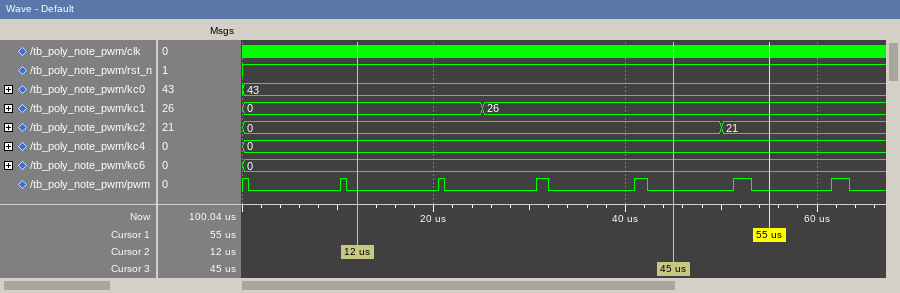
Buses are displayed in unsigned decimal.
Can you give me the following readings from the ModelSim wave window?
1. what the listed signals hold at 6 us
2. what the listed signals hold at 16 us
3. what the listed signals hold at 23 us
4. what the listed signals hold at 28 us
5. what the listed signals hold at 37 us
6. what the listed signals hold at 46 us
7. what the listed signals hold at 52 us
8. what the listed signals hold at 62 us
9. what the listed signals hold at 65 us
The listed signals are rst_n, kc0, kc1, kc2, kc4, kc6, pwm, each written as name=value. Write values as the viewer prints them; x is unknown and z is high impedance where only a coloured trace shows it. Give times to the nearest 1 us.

rst_n=1, kc0=43, kc1=0, kc2=0, kc4=0, kc6=0, pwm=0
rst_n=1, kc0=43, kc1=0, kc2=0, kc4=0, kc6=0, pwm=0
rst_n=1, kc0=43, kc1=0, kc2=0, kc4=0, kc6=0, pwm=0
rst_n=1, kc0=43, kc1=26, kc2=0, kc4=0, kc6=0, pwm=0
rst_n=1, kc0=43, kc1=26, kc2=0, kc4=0, kc6=0, pwm=0
rst_n=1, kc0=43, kc1=26, kc2=0, kc4=0, kc6=0, pwm=0
rst_n=1, kc0=43, kc1=26, kc2=21, kc4=0, kc6=0, pwm=1
rst_n=1, kc0=43, kc1=26, kc2=21, kc4=0, kc6=0, pwm=1
rst_n=1, kc0=43, kc1=26, kc2=21, kc4=0, kc6=0, pwm=0
